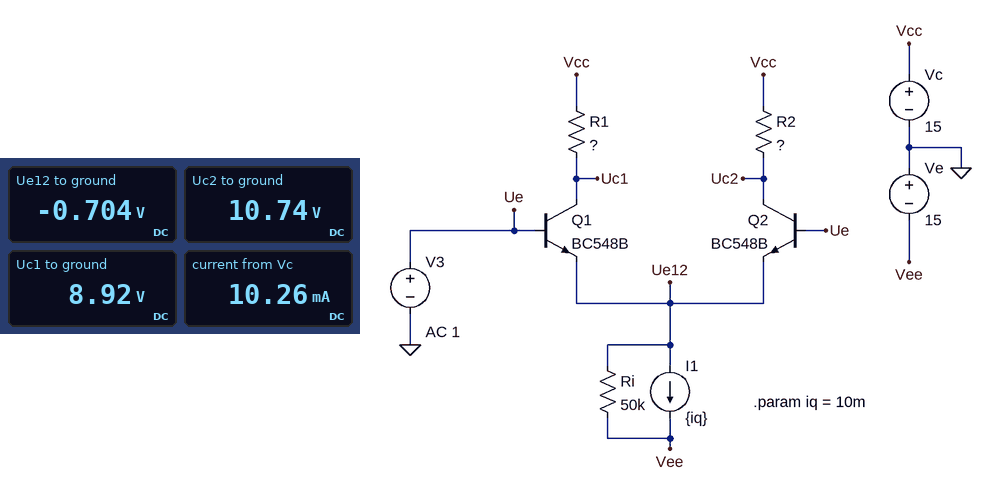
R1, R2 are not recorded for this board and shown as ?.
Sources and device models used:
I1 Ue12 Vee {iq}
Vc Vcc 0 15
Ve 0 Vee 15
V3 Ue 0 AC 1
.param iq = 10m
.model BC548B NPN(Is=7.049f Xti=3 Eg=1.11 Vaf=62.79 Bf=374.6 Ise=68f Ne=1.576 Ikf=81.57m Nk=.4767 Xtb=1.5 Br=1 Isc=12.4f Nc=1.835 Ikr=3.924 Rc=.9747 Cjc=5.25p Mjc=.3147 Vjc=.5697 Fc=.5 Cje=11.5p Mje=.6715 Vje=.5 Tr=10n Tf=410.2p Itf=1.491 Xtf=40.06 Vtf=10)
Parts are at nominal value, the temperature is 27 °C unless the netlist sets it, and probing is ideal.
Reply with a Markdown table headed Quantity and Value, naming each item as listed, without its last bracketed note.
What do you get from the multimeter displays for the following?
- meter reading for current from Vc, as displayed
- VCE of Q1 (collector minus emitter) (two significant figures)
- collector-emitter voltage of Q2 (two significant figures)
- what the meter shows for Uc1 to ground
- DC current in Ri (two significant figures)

| Quantity | Value |
|---|---|
| meter reading for current from Vc, as displayed | 10.26 mA |
| VCE of Q1 (collector minus emitter) | 9.6 V |
| collector-emitter voltage of Q2 | 11 V |
| what the meter shows for Uc1 to ground | 8.92 V |
| DC current in Ri | 290 µA |
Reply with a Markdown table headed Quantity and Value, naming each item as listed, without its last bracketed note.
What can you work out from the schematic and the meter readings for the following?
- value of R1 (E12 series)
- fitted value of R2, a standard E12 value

| Quantity | Value |
|---|---|
| value of R1 | 1.2 kΩ |
| fitted value of R2, a standard E12 value | 820 Ω |
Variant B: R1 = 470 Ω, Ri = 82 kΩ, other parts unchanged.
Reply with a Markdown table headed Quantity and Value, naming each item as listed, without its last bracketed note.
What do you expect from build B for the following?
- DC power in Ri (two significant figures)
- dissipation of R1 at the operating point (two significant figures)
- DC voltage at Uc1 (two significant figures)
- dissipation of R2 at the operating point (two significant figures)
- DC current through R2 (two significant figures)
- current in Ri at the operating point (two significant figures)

| Quantity | Value |
|---|---|
| DC power in Ri | 2.5 mW |
| dissipation of R1 at the operating point | 12 mW |
| DC voltage at Uc1 | 13 V |
| dissipation of R2 at the operating point | 21 mW |
| DC current through R2 | 5.0 mA |
| current in Ri at the operating point | 170 µA |
